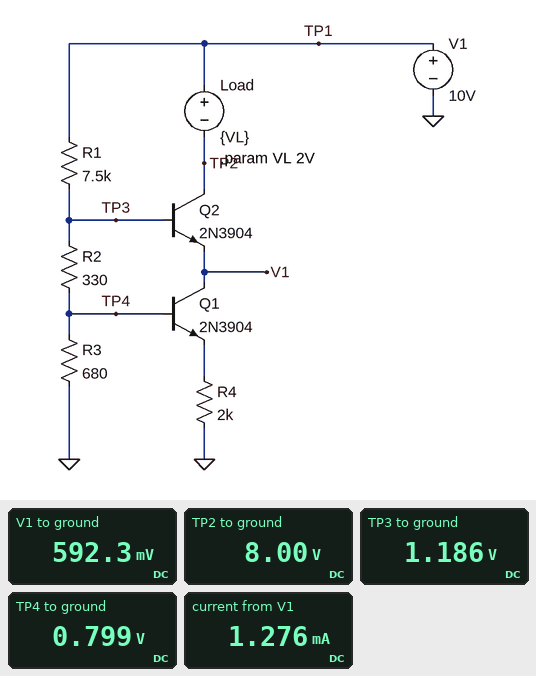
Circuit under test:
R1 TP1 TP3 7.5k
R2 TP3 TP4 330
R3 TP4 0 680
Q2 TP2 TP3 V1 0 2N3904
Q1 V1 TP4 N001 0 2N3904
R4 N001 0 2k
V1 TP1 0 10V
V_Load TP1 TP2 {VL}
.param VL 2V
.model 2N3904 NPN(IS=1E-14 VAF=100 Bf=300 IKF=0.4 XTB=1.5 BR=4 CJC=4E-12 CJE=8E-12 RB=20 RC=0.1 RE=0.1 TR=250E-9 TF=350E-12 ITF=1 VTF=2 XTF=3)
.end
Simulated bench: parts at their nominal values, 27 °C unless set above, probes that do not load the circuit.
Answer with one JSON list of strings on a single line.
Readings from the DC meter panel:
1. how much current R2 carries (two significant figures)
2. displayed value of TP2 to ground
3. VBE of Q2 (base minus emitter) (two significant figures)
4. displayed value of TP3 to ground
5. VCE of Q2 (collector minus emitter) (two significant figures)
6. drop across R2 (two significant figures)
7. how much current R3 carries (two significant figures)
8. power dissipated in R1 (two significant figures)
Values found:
["1.2 mA", "8.00 V", "590 mV", "1.186 V", "7.4 V", "390 mV", "1.2 mA", "10 mW"]
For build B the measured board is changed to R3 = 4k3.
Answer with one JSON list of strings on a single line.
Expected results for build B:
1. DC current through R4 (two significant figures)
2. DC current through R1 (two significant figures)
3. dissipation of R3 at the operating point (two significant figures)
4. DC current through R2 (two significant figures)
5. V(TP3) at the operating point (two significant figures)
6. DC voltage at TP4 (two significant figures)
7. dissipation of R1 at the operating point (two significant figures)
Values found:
["1.4 mA", "830 µA", "2.9 mW", "820 µA", "3.8 V", "3.5 V", "5.1 mW"]
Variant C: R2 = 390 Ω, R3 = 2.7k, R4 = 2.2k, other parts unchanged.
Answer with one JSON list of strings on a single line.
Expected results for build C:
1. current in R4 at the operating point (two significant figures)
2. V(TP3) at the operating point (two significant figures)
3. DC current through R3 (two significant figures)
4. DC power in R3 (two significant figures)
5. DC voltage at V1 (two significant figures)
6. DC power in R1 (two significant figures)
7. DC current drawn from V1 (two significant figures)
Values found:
["860 µA", "2.9 V", "940 µA", "2.4 mW", "2.3 V", "6.7 mW", "1.8 mA"]
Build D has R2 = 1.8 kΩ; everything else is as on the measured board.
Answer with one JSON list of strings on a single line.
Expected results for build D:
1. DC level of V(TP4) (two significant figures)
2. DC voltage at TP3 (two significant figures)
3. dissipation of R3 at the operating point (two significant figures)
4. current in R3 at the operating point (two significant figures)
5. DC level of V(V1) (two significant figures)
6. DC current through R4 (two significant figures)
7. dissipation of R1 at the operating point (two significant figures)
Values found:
["680 mV", "2.5 V", "680 µW", "1.0 mA", "1.9 V", "52 µA", "7.5 mW"]
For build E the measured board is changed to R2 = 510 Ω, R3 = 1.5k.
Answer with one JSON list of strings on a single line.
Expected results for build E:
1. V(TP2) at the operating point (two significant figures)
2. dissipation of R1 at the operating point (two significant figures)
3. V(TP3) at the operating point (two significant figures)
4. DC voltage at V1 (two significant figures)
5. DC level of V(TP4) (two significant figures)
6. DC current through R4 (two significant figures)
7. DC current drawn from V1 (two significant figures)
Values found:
["8.0 V", "8.3 mW", "2.1 V", "1.5 V", "1.6 V", "470 µA", "1.5 mA"]
